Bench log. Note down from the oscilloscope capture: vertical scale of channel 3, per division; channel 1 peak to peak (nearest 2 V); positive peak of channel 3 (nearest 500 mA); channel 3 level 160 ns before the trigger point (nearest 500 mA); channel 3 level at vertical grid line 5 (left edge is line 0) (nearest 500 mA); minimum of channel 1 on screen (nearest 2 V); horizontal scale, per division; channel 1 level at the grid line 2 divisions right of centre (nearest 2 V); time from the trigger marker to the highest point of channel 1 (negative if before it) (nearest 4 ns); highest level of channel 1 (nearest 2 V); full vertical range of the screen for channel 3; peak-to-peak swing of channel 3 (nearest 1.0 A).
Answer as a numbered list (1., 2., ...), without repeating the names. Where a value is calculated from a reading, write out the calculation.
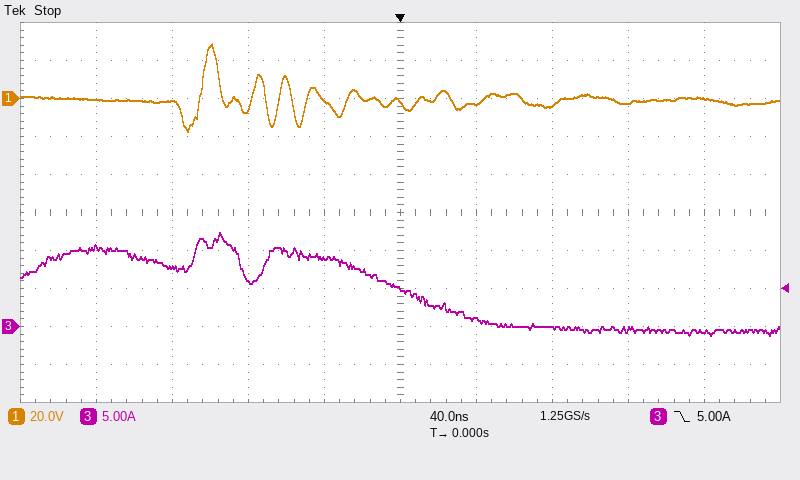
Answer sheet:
1. 5 A
2. 28 V − (-18 V) = 46 V
3. 12.5 A
4. 10.5 A
5. 5.0 A
6. -18 V
7. 40 ns
8. -4 V
9. -100 ns
10. 28 V
11. 50 A
12. 14.0 A
